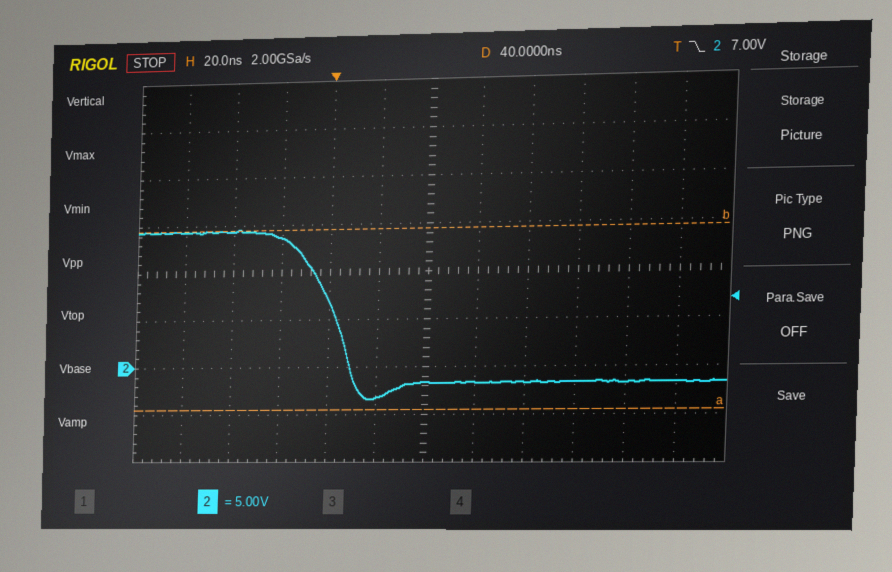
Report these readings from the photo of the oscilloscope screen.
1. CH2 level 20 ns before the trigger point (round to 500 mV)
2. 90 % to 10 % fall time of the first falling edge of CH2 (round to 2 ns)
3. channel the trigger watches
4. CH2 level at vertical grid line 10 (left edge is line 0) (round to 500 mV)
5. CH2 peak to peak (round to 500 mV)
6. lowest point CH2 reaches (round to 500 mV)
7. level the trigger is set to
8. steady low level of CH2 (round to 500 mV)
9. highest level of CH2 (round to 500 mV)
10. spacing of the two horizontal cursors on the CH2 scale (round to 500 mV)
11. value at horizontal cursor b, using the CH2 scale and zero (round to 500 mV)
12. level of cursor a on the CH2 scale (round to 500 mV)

13.5 V
24 ns
CH2
-1.5 V
18.0 V
-3.5 V
7.00 V
-1.5 V
14.5 V
19.0 V
14.5 V
-4.5 V
